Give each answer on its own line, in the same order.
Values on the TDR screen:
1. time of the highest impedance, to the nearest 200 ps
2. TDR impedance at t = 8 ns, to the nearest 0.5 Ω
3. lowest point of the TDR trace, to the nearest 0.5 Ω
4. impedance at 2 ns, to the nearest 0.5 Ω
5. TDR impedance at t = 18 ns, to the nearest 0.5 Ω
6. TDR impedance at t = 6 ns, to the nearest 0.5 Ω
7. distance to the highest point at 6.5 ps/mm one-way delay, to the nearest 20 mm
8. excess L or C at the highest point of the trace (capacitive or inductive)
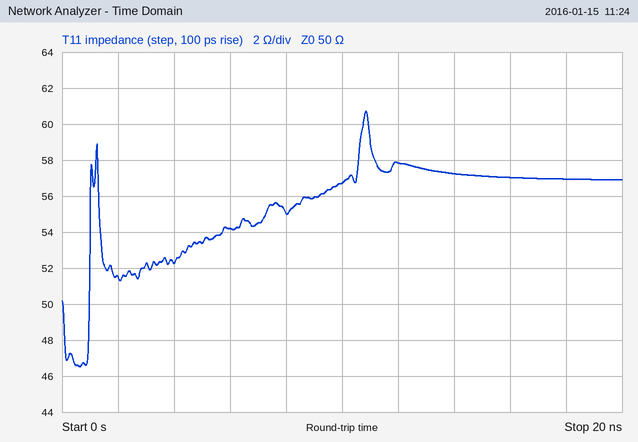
10.8 ns
55.0 Ω
46.5 Ω
51.5 Ω
57.0 Ω
54.0 Ω
840 mm
inductive
